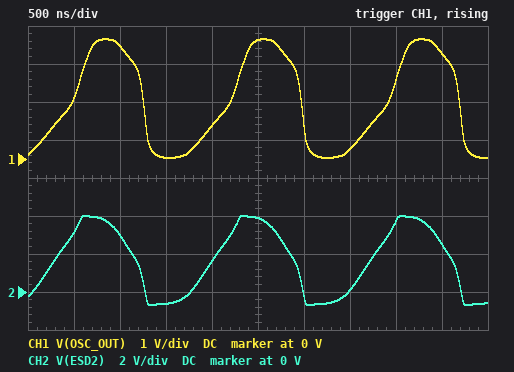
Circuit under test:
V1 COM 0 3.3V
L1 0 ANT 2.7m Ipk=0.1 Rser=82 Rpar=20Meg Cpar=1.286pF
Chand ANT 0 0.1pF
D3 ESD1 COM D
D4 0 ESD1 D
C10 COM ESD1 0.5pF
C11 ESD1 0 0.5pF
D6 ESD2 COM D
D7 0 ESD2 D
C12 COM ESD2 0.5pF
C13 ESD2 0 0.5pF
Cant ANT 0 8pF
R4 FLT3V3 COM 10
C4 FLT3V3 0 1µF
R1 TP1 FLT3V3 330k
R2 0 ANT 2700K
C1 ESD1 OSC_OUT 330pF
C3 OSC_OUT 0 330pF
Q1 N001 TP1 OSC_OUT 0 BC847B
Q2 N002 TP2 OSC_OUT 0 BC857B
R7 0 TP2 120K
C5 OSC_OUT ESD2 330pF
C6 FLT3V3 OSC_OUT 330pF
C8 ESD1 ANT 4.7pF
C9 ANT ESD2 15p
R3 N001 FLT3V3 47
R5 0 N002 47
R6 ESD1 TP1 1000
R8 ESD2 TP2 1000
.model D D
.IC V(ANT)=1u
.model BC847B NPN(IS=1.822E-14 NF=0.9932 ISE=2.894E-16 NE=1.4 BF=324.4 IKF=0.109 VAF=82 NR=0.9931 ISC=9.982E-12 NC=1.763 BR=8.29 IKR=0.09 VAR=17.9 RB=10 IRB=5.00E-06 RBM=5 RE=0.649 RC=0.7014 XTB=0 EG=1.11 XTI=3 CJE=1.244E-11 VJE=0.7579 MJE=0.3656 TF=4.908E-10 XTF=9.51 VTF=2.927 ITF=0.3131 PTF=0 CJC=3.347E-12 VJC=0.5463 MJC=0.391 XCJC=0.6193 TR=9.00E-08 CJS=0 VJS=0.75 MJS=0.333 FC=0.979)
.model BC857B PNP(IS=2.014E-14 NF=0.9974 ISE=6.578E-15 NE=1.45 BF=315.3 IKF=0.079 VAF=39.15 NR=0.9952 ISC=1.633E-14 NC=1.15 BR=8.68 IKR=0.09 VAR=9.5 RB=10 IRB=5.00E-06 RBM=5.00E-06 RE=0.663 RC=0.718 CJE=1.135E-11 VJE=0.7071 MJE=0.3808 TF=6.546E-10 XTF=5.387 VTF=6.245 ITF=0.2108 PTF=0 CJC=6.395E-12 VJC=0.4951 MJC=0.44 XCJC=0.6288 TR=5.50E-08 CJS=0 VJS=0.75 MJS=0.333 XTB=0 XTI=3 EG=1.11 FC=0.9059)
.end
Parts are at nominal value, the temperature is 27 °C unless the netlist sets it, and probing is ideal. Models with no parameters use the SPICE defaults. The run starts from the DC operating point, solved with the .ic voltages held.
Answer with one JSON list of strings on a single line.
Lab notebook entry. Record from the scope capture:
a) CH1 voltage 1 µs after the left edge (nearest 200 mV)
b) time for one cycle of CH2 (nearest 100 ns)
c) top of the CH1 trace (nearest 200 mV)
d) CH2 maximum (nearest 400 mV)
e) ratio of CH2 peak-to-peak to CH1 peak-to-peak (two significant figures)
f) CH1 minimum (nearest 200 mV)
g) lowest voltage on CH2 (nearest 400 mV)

["3.0 V", "1.7 µs", "3.2 V", "4.0 V", "1.5", "0 V", "-800 mV"]
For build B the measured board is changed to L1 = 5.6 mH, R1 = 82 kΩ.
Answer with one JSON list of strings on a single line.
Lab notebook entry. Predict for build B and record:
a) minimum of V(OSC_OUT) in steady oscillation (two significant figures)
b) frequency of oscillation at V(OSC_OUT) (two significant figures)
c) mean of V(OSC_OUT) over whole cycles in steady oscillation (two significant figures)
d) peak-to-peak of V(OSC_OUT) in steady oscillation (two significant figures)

["16 mV", "410 kHz", "1.6 V", "3.2 V"]
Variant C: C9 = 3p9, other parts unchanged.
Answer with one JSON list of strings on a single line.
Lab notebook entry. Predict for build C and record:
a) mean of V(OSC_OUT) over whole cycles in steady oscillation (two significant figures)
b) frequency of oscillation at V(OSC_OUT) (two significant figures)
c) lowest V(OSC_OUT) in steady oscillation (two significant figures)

["1.6 V", "730 kHz", "100 mV"]
